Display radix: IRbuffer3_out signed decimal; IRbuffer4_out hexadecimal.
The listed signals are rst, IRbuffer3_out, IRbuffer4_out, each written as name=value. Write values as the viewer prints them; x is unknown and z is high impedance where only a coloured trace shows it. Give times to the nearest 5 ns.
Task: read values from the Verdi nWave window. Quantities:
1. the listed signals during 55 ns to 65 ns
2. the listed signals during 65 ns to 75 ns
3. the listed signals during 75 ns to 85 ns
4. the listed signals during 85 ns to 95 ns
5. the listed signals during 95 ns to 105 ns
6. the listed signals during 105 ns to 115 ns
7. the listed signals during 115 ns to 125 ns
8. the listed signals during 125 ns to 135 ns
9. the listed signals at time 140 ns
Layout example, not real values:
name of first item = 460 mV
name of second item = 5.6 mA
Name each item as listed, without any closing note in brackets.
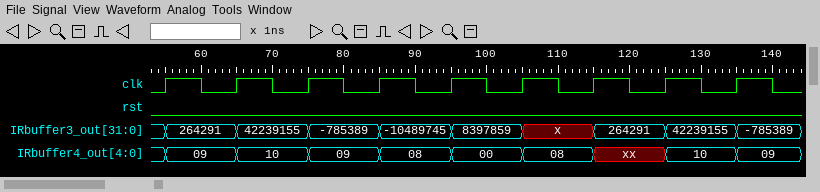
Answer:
the listed signals during 55 ns to 65 ns = rst=0, IRbuffer3_out=264291, IRbuffer4_out=09
the listed signals during 65 ns to 75 ns = rst=0, IRbuffer3_out=42239155, IRbuffer4_out=10
the listed signals during 75 ns to 85 ns = rst=0, IRbuffer3_out=-785389, IRbuffer4_out=09
the listed signals during 85 ns to 95 ns = rst=0, IRbuffer3_out=-10489745, IRbuffer4_out=08
the listed signals during 95 ns to 105 ns = rst=0, IRbuffer3_out=8397859, IRbuffer4_out=00
the listed signals during 105 ns to 115 ns = rst=0, IRbuffer3_out=x, IRbuffer4_out=08
the listed signals during 115 ns to 125 ns = rst=0, IRbuffer3_out=264291, IRbuffer4_out=xx
the listed signals during 125 ns to 135 ns = rst=0, IRbuffer3_out=42239155, IRbuffer4_out=10
the listed signals at time 140 ns = rst=0, IRbuffer3_out=-785389, IRbuffer4_out=09
